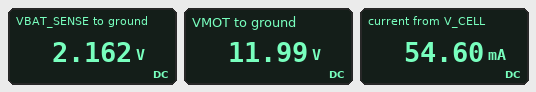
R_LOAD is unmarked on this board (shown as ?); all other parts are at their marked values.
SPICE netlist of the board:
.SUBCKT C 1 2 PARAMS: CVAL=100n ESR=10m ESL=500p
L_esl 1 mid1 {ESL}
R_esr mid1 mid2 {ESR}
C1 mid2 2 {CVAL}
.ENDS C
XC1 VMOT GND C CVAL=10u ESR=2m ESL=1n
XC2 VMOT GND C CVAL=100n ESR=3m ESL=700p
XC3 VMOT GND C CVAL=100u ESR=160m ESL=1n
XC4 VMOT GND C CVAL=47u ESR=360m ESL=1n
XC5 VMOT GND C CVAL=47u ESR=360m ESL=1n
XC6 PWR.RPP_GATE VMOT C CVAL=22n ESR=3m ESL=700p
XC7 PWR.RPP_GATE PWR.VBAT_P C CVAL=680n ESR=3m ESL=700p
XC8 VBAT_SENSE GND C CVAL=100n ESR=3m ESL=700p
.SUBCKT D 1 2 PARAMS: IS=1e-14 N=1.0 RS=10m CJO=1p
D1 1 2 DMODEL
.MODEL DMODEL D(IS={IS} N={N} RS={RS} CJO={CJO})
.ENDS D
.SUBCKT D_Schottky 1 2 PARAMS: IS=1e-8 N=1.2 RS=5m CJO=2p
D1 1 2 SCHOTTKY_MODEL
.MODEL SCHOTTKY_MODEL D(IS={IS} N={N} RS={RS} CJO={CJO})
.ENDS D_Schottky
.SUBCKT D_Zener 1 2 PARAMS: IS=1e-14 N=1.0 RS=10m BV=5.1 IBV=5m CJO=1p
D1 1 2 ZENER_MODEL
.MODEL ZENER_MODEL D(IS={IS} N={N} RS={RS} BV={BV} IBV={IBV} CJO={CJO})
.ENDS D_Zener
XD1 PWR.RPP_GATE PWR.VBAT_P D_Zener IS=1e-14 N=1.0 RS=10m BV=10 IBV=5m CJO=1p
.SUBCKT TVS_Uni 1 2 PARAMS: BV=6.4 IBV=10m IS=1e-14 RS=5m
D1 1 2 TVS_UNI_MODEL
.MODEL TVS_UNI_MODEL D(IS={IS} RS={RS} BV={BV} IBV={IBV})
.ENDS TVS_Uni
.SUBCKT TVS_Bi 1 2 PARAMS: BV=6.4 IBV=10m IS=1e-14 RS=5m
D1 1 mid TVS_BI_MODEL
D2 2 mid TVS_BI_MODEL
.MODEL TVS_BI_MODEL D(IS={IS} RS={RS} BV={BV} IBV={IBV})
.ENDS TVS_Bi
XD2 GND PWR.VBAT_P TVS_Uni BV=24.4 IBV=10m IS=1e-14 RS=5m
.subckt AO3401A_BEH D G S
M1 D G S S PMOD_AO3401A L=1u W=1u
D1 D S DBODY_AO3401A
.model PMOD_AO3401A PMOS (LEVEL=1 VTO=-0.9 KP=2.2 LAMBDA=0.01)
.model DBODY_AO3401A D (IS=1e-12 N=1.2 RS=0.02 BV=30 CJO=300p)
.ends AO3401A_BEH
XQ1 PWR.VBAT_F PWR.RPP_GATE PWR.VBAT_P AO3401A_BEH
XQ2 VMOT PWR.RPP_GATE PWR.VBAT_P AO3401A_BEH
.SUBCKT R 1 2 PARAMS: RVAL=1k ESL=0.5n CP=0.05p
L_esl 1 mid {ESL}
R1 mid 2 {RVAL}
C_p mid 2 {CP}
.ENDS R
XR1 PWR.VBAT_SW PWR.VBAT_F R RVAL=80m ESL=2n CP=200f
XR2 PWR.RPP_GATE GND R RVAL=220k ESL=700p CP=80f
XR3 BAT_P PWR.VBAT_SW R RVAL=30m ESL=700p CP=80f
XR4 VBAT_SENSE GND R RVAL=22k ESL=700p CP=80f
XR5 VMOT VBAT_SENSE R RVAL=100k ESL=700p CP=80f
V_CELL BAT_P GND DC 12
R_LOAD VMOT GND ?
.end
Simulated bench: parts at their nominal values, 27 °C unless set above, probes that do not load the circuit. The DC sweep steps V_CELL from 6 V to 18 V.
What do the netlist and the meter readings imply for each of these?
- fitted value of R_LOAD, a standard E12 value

220 Ω
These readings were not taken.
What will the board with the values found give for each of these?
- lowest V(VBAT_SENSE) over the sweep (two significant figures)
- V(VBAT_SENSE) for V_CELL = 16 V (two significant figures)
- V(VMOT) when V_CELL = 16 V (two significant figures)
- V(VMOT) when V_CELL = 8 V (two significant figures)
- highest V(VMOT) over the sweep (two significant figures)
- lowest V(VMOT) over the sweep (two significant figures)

1.1 V
2.9 V
16 V
8.0 V
18 V
6.0 V
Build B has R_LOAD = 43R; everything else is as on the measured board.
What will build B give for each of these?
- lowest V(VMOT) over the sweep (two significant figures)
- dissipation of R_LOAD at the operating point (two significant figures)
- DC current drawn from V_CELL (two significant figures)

6.0 V
3.3 W
280 mA
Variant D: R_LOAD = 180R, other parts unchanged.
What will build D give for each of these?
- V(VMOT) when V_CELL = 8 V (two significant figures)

8.0 V
